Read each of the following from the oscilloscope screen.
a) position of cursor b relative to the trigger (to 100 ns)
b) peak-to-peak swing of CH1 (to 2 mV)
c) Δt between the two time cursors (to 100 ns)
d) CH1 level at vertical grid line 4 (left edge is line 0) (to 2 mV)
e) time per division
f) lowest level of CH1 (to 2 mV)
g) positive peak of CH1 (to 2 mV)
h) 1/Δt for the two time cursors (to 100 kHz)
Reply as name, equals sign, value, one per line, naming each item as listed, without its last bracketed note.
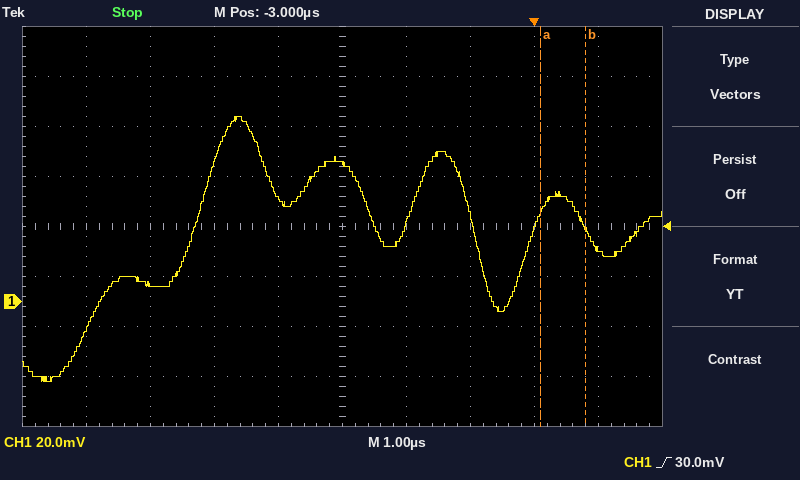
position of cursor b relative to the trigger = +800 ns
peak-to-peak swing of CH1 = 106 mV
Δt between the two time cursors = 700 ns
CH1 level at vertical grid line 4 (left edge is line 0) = 42 mV
time per division = 1 µs
lowest level of CH1 = -32 mV
positive peak of CH1 = 74 mV
1/Δt for the two time cursors = 1.4 MHz
